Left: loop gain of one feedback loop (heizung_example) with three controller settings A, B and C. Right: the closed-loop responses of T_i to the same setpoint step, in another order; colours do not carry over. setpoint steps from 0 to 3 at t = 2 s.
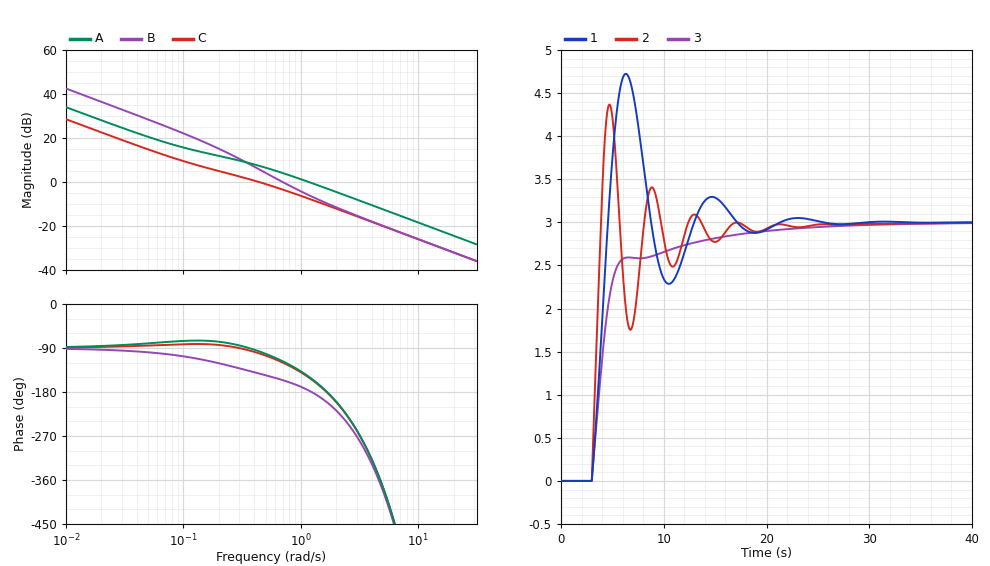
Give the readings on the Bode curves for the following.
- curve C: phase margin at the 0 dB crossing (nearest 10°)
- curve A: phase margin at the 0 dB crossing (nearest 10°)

80°
30°
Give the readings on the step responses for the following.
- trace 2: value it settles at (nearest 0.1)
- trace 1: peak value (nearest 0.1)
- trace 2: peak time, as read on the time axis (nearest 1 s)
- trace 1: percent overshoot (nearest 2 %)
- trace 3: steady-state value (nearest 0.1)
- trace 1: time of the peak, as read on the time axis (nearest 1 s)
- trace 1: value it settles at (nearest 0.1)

3.0
4.7
5 s
58 %
3.0
6 s
3.0
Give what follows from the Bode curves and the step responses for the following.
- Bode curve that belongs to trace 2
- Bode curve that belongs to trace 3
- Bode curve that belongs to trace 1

A
C
B
